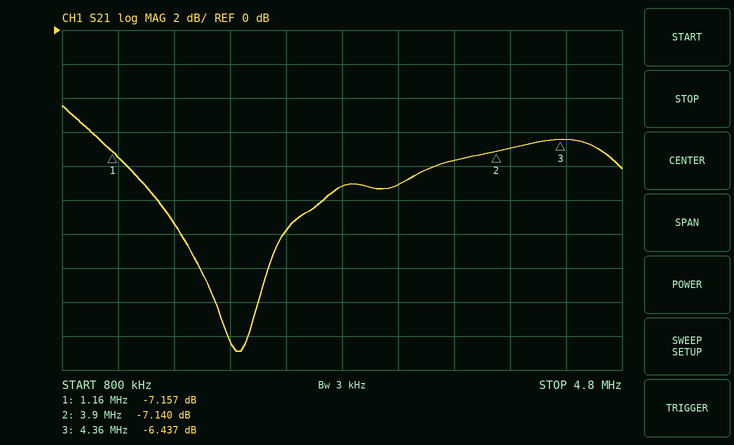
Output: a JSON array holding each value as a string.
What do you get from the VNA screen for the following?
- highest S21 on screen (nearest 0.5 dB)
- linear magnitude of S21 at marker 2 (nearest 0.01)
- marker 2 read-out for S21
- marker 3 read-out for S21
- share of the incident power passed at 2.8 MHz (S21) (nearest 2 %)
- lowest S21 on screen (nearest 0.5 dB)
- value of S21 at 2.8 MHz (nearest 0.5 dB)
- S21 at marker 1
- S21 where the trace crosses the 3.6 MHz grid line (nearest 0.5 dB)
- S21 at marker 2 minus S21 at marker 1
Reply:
["-4.5 dB", "0.44", "-7.140 dB", "-6.437 dB", "12 %", "-19.0 dB", "-9.0 dB", "-7.157 dB", "-7.5 dB", "0.017 dB"]
